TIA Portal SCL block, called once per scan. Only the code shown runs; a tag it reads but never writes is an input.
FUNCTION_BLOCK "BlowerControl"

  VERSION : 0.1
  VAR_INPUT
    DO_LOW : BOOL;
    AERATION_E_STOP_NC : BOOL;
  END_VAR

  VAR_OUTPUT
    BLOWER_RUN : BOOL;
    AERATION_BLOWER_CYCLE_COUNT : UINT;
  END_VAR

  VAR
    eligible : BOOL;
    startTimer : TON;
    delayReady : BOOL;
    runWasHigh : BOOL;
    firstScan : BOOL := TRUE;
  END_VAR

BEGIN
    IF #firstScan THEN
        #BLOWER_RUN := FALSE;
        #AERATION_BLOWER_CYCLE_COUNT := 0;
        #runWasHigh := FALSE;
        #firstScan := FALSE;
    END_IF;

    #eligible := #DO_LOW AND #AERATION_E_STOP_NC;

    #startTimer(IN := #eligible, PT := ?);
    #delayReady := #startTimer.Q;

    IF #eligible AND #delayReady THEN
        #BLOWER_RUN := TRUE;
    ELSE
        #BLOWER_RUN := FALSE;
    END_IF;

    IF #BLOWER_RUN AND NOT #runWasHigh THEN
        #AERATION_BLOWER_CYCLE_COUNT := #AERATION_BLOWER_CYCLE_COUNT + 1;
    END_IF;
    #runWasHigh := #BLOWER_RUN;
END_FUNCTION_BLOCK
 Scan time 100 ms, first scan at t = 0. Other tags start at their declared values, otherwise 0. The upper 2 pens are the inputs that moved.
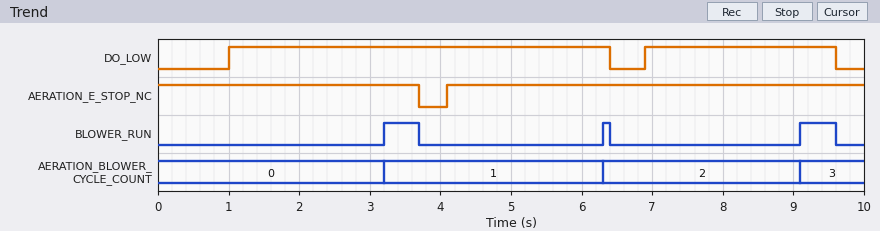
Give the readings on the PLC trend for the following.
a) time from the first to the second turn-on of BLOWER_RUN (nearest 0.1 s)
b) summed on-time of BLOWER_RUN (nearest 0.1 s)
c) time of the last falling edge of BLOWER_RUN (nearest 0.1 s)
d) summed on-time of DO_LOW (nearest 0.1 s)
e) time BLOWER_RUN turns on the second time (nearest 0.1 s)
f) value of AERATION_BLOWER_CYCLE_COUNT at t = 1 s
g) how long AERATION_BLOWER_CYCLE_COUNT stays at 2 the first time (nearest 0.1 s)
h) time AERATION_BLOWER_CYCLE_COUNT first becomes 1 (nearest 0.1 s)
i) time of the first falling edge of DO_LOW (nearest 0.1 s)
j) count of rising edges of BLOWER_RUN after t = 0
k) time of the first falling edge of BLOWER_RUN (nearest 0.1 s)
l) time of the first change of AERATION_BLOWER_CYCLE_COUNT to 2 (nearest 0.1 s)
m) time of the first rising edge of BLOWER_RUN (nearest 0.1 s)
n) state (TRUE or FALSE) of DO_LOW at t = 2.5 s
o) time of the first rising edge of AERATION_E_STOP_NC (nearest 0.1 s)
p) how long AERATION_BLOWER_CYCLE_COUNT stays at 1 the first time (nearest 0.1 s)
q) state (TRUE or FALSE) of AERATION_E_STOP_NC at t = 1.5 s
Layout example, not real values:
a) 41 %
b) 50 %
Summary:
a) 3.1 s
b) 1.1 s
c) 9.6 s
d) 8.1 s
e) 6.3 s
f) 0
g) 2.8 s
h) 3.2 s
i) 6.4 s
j) 3
k) 3.7 s
l) 6.3 s
m) 3.2 s
n) TRUE
o) 4.1 s
p) 3.1 s
q) TRUE
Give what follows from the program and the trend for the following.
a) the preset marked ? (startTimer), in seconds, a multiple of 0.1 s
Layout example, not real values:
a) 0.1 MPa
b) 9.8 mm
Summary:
a) 2.2 s
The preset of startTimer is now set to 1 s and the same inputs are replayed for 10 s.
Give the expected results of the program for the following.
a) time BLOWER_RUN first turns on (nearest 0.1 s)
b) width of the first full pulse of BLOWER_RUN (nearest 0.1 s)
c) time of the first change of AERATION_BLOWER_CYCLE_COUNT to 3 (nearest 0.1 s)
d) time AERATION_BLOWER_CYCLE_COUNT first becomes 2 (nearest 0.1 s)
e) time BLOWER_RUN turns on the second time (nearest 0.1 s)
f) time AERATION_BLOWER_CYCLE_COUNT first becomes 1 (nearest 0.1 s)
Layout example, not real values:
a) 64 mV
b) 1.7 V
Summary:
a) 2.0 s
b) 1.7 s
c) 7.9 s
d) 5.1 s
e) 5.1 s
f) 2.0 s
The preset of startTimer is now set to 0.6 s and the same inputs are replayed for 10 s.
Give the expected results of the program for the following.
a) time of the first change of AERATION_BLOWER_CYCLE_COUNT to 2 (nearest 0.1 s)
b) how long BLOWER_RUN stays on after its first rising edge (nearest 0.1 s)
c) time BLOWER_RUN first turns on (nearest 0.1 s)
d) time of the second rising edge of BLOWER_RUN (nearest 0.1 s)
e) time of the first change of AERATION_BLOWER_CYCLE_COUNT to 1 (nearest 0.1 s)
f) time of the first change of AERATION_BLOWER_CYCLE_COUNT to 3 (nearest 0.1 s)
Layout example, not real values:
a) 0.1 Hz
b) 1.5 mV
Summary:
a) 4.7 s
b) 2.1 s
c) 1.6 s
d) 4.7 s
e) 1.6 s
f) 7.5 s
